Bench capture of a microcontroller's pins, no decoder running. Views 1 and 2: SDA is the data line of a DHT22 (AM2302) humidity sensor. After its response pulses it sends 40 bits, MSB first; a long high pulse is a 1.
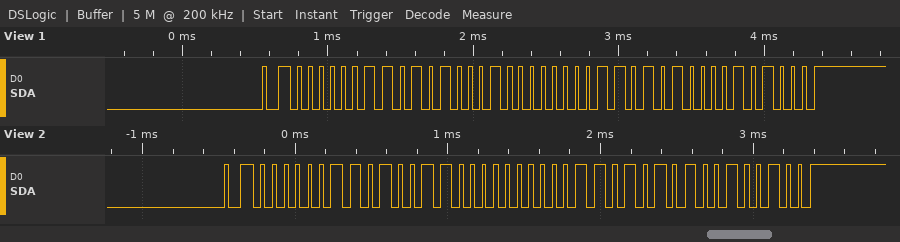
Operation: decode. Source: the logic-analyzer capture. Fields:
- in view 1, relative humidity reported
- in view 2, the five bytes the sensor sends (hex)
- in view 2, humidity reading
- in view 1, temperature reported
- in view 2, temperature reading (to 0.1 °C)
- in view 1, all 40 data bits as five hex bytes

84.9 %
03 4C 00 D5 24
84.4 %
21.2 °C
21.3 °C
03 51 00 D4 28
